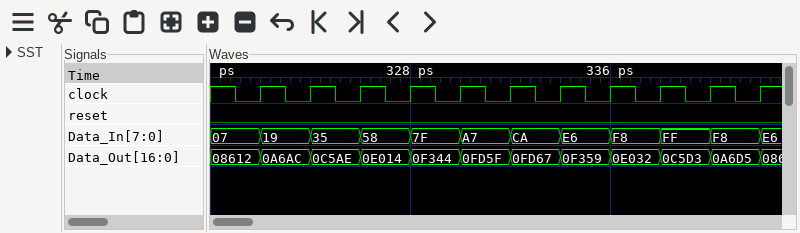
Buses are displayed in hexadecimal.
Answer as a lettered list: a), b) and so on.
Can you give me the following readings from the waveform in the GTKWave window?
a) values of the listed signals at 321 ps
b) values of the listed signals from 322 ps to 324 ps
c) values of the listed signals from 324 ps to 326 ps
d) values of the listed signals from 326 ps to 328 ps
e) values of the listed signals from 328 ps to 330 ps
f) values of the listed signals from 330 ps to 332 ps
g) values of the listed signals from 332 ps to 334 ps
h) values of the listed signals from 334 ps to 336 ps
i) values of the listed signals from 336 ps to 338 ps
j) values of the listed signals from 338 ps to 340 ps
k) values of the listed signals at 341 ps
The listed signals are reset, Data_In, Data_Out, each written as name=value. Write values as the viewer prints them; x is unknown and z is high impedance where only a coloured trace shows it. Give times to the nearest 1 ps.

a) reset=0, Data_In=07, Data_Out=08612
b) reset=0, Data_In=19, Data_Out=0A6AC
c) reset=0, Data_In=35, Data_Out=0C5AE
d) reset=0, Data_In=58, Data_Out=0E014
e) reset=0, Data_In=7F, Data_Out=0F344
f) reset=0, Data_In=A7, Data_Out=0FD5F
g) reset=0, Data_In=CA, Data_Out=0FD67
h) reset=0, Data_In=E6, Data_Out=0F359
i) reset=0, Data_In=F8, Data_Out=0E032
j) reset=0, Data_In=FF, Data_Out=0C5D3
k) reset=0, Data_In=F8, Data_Out=0A6D5
